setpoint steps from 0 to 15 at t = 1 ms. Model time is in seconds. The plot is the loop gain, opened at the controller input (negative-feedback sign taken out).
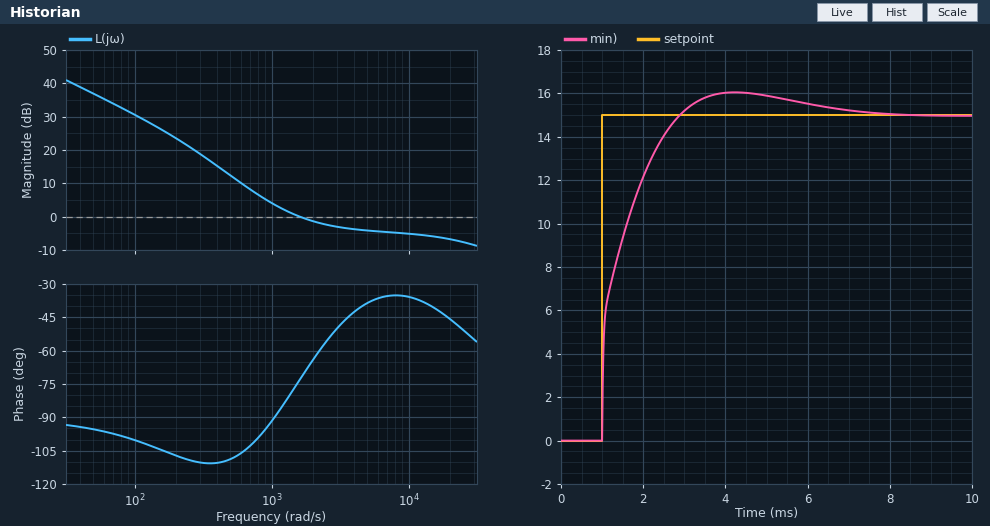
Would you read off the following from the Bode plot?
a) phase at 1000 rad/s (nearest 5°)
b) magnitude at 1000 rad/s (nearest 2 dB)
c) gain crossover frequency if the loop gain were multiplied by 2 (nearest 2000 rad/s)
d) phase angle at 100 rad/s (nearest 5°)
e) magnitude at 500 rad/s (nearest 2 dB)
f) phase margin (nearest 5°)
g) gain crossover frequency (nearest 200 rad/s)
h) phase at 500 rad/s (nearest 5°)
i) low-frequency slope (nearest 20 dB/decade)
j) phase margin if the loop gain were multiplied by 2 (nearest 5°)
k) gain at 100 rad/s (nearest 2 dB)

-90°
4 dB
16000 rad/s
-100°
12 dB
105°
1600 rad/s
-110°
-20 dB/decade
140°
30 dB
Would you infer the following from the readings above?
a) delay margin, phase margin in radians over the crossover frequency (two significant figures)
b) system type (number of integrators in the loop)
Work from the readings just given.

0.0011 s
1
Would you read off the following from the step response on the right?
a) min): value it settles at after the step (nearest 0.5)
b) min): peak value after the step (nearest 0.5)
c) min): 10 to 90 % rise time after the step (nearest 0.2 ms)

15.0
16.0
1.4 ms
